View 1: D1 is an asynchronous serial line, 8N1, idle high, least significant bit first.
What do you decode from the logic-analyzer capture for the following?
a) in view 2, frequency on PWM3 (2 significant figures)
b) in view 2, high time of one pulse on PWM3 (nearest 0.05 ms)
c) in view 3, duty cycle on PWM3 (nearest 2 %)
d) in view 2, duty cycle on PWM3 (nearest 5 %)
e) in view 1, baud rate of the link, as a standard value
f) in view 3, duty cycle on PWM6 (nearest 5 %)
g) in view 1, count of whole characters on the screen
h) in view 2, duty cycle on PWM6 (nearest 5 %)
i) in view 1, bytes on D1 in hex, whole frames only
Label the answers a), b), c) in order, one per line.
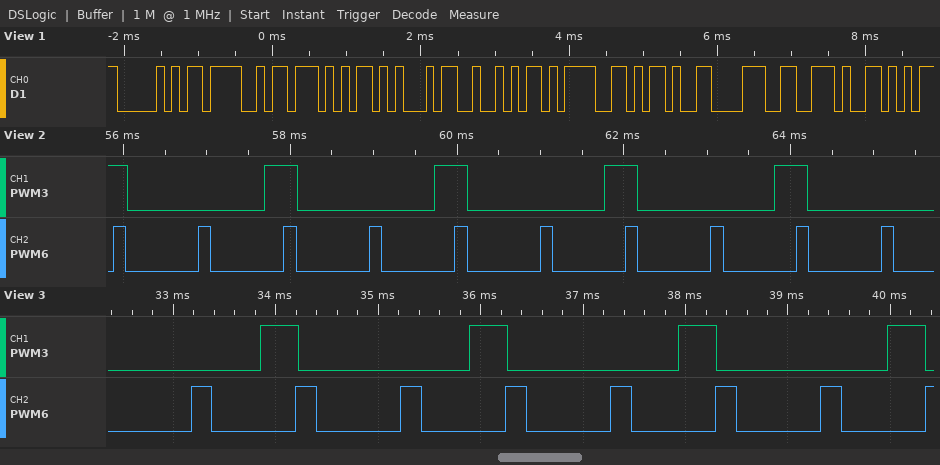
a) 490 Hz
b) 0.40 ms
c) 18 %
d) 20 %
e) 9600 baud
f) 20 %
g) 9
h) 15 %
i) 0x50 0x4F 0x57 0x45 0x52 0x3D 0x2D 0x38 0x2E
